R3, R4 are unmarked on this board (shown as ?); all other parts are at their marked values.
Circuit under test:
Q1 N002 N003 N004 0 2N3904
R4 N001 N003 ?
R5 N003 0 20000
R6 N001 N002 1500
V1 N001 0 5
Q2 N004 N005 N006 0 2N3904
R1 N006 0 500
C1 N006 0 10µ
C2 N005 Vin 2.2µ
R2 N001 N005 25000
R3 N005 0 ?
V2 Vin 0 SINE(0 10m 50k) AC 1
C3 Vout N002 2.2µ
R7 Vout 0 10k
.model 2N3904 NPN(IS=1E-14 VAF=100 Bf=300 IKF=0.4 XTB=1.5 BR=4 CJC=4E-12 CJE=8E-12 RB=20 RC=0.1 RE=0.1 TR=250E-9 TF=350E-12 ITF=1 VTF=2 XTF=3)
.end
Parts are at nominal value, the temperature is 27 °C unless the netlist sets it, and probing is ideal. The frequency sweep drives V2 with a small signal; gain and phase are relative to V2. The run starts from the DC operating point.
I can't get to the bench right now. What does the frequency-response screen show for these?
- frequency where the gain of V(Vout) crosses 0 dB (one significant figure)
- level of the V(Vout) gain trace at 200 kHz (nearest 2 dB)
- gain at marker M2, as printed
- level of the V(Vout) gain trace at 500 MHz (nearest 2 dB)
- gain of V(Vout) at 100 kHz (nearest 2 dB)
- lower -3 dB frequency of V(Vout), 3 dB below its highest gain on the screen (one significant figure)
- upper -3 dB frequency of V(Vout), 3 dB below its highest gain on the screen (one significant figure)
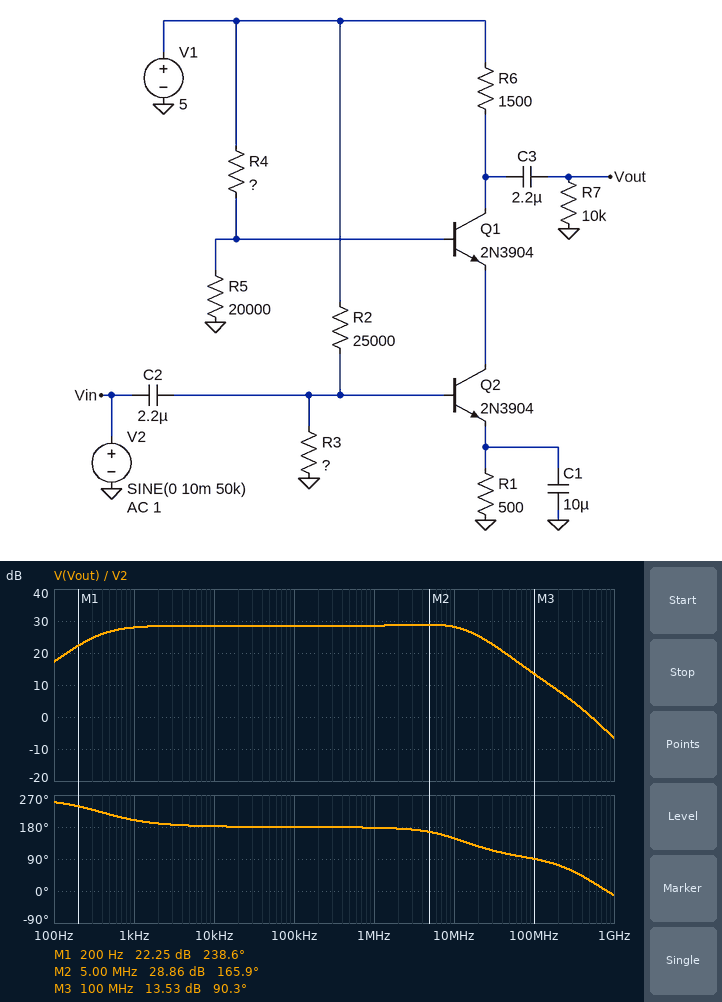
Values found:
500 MHz
28 dB
28.86 dB
0 dB
28 dB
400 Hz
20 MHz
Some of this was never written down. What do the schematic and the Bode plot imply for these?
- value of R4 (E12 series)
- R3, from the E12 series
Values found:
33 kΩ
5.6 kΩ
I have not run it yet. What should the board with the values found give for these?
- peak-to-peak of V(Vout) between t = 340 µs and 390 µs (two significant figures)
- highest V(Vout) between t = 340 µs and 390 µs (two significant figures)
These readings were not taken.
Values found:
540 mV
230 mV
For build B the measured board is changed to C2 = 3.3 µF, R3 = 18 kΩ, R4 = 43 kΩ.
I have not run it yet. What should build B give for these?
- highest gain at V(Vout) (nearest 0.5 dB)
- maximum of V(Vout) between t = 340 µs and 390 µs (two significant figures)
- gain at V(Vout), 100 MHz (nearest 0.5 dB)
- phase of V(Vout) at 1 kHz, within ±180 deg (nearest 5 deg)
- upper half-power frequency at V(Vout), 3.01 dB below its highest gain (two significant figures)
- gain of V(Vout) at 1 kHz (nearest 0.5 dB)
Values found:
32.0 dB
470 mV
-9.0 dB
-130 deg
350 kHz
29.5 dB
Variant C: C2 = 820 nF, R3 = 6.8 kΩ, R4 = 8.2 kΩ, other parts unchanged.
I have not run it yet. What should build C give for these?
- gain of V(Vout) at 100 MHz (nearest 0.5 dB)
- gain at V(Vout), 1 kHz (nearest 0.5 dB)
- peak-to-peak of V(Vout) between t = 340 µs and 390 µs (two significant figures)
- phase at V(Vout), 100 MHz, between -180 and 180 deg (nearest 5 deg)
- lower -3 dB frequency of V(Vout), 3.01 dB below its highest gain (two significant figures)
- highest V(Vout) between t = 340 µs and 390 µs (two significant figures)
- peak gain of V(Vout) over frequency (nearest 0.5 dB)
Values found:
19.0 dB
31.0 dB
810 mV
95 deg
550 Hz
350 mV
32.0 dB
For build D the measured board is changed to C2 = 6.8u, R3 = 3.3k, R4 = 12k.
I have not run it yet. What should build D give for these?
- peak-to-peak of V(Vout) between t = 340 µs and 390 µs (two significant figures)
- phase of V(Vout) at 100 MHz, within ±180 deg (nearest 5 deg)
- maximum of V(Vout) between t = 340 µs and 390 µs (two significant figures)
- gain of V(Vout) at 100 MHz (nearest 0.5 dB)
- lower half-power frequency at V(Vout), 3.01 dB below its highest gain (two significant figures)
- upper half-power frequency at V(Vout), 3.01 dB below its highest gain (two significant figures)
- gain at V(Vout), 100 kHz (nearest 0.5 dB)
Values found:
34 mV
75 deg
14 mV
-2.0 dB
33 Hz
7.3 MHz
4.5 dB
